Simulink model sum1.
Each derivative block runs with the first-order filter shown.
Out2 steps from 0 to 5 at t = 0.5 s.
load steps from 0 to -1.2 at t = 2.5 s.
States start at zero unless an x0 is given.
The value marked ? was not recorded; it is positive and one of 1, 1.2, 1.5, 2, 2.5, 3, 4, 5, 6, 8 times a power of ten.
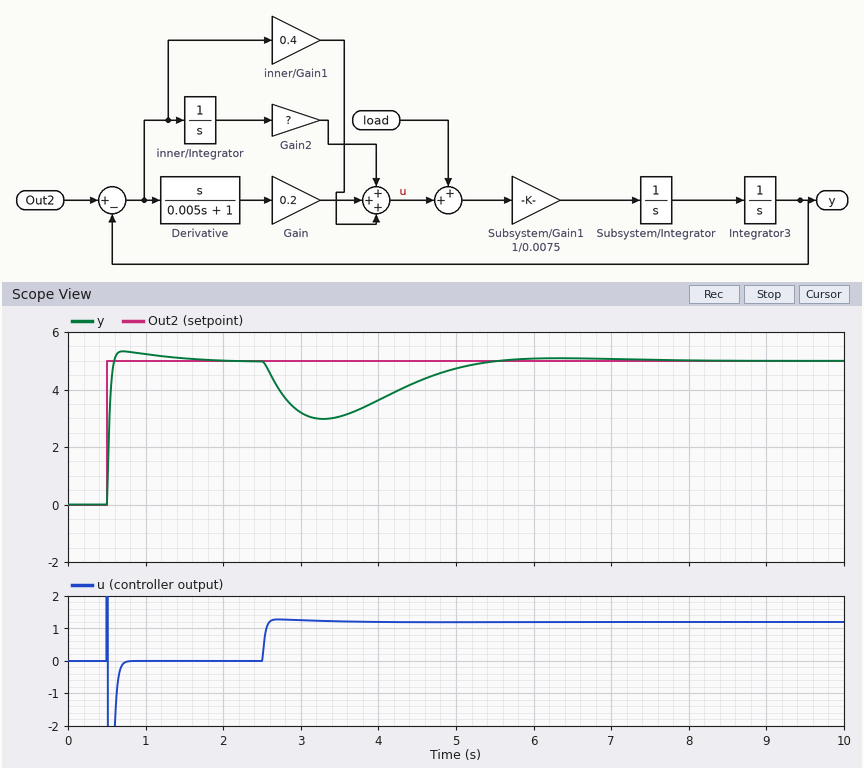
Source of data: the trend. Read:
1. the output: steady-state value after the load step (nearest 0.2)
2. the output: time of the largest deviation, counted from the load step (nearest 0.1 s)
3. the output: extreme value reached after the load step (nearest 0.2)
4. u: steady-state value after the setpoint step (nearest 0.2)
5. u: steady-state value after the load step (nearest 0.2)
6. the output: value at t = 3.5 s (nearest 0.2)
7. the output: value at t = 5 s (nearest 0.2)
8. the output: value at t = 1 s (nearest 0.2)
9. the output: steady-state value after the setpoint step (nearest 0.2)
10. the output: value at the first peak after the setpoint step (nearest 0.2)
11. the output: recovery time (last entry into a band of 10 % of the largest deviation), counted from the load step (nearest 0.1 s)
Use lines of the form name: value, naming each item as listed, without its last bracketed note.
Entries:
the output: steady-state value after the load step: 5.0
the output: time of the largest deviation, counted from the load step: 0.8 s
the output: extreme value reached after the load step: 3.0
u: steady-state value after the setpoint step: 0.0
u: steady-state value after the load step: 1.2
the output: value at t = 3.5 s: 3.0
the output: value at t = 5 s: 4.8
the output: value at t = 1 s: 5.2
the output: steady-state value after the setpoint step: 5.0
the output: value at the first peak after the setpoint step: 5.4
the output: recovery time (last entry into a band of 10 % of the largest deviation), counted from the load step: 2.6 s
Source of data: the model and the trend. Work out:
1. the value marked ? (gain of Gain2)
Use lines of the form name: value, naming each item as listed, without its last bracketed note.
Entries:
the value marked ?: 0.4
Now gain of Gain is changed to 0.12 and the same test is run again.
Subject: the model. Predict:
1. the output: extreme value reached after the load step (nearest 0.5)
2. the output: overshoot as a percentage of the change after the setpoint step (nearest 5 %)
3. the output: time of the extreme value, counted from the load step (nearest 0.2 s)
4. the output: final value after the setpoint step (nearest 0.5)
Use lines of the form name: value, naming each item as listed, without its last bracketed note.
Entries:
the output: extreme value reached after the load step: 2.5
the output: overshoot as a percentage of the change after the setpoint step: 15 %
the output: time of the extreme value, counted from the load step: 0.6 s
the output: final value after the setpoint step: 5.0
